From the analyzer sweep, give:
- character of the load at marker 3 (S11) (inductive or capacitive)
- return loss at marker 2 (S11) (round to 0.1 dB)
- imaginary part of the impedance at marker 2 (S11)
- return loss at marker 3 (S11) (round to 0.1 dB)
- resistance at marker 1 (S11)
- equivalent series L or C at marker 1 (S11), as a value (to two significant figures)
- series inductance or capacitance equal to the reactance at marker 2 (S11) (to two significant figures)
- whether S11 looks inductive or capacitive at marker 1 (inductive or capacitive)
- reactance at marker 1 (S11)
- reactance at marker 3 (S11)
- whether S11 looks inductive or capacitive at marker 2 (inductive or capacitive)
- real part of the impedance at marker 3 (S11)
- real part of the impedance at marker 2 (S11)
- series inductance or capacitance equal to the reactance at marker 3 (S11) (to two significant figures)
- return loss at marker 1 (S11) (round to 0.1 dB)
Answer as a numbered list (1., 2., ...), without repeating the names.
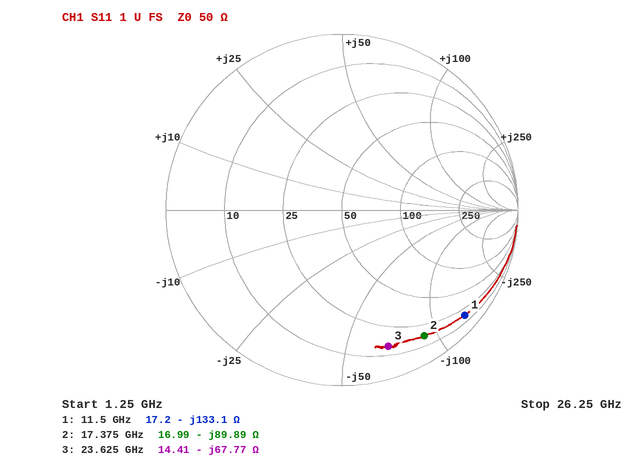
1. capacitive
2. 1.4 dB
3. -89.89 Ω
4. 1.7 dB
5. 17.2 Ω
6. 100 fF
7. 100 fF
8. capacitive
9. -133.1 Ω
10. -67.77 Ω
11. capacitive
12. 14.41 Ω
13. 16.99 Ω
14. 99 fF
15. 0.7 dB
